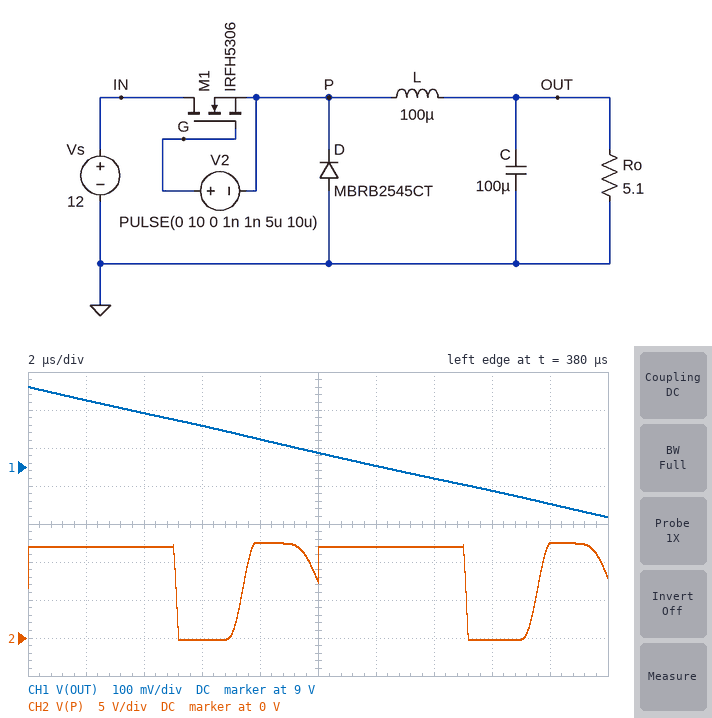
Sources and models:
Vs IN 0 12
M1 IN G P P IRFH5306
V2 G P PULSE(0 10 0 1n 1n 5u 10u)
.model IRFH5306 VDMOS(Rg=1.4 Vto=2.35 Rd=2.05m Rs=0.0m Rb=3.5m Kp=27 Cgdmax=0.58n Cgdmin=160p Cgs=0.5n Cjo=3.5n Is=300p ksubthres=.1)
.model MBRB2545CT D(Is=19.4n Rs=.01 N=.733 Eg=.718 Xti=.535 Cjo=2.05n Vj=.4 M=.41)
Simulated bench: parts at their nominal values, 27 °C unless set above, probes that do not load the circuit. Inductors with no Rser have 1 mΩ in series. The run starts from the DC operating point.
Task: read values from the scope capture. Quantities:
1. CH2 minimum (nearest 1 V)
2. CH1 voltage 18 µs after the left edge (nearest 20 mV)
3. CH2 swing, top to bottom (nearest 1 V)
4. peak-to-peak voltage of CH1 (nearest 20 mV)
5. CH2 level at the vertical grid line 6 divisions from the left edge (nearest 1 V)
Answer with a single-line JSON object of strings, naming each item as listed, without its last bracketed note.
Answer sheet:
{"CH2 minimum": "0 V", "CH1 voltage 18 µs after the left edge": "8.90 V", "CH2 swing, top to bottom": "13 V", "peak-to-peak voltage of CH1": "340 mV", "CH2 level at the vertical grid line 6 divisions from the left edge": "12 V"}
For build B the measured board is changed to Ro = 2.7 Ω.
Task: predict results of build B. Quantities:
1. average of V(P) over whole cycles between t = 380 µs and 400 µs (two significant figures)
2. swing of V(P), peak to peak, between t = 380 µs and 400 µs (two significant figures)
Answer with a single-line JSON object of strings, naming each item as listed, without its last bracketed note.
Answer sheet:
{"average of V(P) over whole cycles between t = 380 µs and 400 µs": "5.8 V", "swing of V(P), peak to peak, between t = 380 µs and 400 µs": "12 V"}
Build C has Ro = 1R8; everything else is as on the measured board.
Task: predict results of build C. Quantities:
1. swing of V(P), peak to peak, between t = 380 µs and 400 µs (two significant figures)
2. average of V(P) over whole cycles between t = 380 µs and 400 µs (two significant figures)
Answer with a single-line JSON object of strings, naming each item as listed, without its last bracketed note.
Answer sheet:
{"swing of V(P), peak to peak, between t = 380 µs and 400 µs": "12 V", "average of V(P) over whole cycles between t = 380 µs and 400 µs": "5.8 V"}
